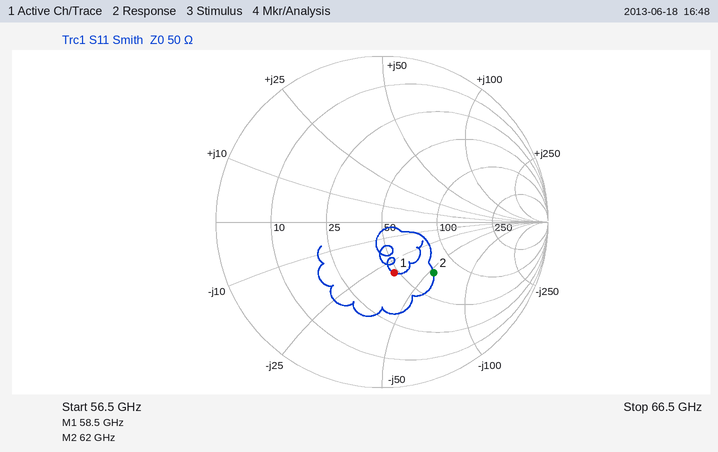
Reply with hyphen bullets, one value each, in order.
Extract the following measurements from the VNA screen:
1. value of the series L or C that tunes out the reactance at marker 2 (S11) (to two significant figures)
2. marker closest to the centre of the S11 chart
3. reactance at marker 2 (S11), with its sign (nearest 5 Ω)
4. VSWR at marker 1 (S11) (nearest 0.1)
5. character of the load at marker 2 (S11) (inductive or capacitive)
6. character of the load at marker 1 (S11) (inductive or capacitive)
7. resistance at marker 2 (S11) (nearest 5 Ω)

- 140 pH
- marker 1
- -55 Ω
- 1.9
- capacitive
- capacitive
- 70 Ω
